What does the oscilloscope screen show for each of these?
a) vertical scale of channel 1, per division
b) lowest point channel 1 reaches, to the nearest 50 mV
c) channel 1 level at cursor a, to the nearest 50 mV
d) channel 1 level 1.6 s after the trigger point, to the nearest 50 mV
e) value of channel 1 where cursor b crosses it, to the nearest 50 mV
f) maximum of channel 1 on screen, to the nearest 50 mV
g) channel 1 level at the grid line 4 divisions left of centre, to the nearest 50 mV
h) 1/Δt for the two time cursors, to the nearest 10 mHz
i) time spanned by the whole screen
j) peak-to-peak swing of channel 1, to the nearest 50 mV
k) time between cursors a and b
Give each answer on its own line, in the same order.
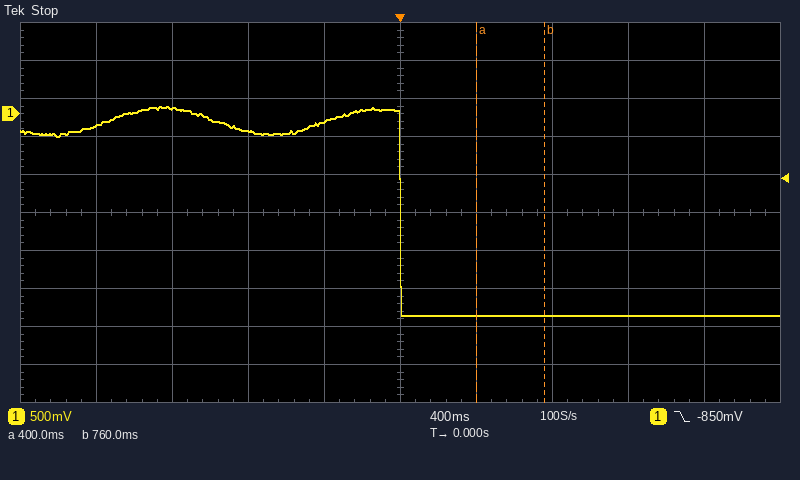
500 mV
-2.65 V
-2.65 V
-2.65 V
-2.65 V
100 mV
-150 mV
2.78 Hz
4 s
2.75 V
360 ms
